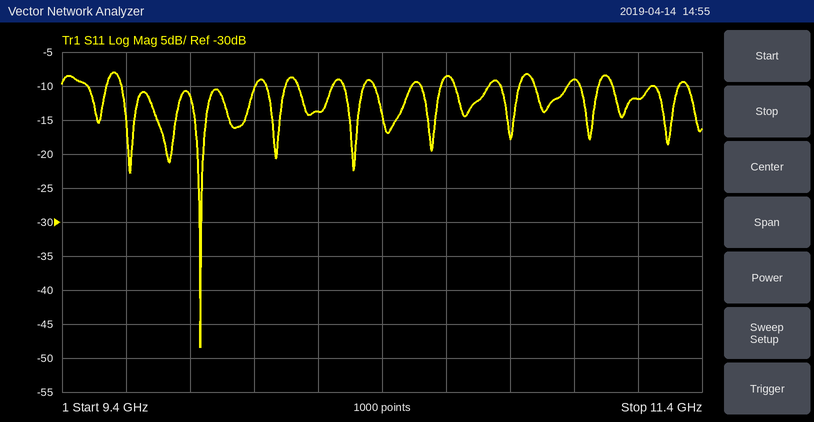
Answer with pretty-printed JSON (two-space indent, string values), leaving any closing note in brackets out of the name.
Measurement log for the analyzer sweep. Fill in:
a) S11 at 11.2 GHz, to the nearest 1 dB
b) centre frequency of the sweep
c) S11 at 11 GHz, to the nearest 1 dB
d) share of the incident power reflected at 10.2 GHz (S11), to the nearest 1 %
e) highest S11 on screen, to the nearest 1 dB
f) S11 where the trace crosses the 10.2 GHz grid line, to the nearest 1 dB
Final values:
{
  "S11 at 11.2 GHz, to the nearest 1 dB": "-12 dB",
  "centre frequency of the sweep": "10.4 GHz",
  "S11 at 11 GHz, to the nearest 1 dB": "-9 dB",
  "share of the incident power reflected at 10.2 GHz (S11), to the nearest 1 %": "4 %",
  "highest S11 on screen, to the nearest 1 dB": "-8 dB",
  "S11 where the trace crosses the 10.2 GHz grid line, to the nearest 1 dB": "-14 dB"
}
